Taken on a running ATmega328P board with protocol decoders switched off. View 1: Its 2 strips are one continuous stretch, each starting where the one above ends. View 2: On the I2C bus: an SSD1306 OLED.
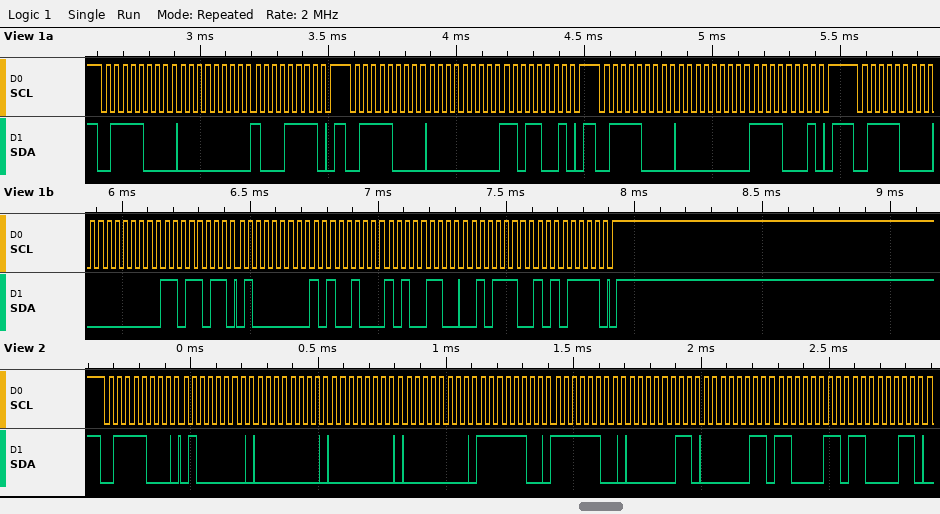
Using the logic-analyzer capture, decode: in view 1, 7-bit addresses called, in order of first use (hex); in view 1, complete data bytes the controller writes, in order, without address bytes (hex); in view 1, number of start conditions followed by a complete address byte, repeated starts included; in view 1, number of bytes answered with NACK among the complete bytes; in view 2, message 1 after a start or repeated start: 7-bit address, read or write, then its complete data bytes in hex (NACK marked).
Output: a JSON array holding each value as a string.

["0x3C", "00 8F 00 D9 00 F1 00 DB 40 A4 A6 2E AF", "4", "0", "0x3C write: 40 00 00 00 FC FC 03 03 C3 C3"]
